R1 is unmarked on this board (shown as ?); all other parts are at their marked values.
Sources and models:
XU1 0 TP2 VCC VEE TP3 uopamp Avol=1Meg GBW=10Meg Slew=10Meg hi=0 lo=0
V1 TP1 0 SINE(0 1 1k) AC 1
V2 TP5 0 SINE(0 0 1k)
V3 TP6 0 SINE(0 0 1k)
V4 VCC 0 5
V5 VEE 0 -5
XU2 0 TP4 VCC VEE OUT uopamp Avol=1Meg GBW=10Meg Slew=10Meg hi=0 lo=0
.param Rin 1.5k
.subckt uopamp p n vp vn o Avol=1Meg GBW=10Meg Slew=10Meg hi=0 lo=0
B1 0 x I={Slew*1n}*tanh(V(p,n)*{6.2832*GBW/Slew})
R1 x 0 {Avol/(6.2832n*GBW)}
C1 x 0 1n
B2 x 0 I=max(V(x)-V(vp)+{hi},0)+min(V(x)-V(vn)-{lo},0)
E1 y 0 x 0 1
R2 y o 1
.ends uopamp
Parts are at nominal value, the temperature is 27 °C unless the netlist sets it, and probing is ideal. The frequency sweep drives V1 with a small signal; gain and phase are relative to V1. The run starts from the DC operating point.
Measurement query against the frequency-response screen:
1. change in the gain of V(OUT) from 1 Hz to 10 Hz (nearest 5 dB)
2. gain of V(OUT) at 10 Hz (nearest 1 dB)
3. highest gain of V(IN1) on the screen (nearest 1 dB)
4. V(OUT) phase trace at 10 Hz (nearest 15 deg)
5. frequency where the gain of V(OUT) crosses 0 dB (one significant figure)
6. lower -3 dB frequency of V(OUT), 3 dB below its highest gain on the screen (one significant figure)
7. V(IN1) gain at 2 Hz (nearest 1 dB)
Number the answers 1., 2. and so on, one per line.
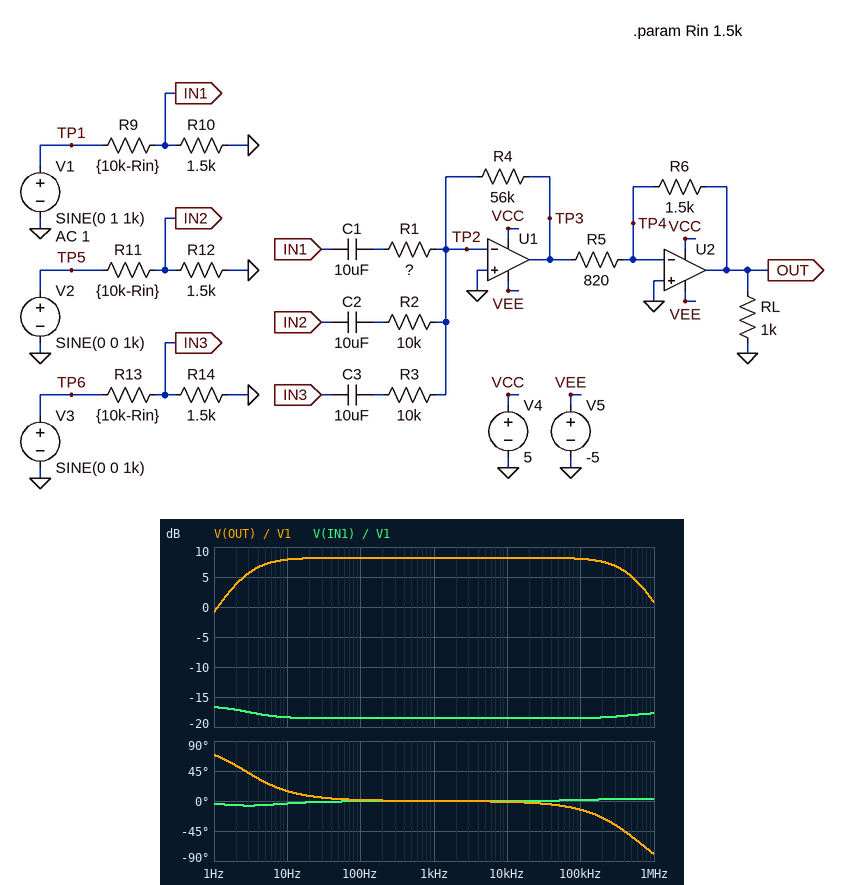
1. 10 dB
2. 8 dB
3. -17 dB
4. 15 deg
5. 1 Hz
6. 3 Hz
7. -17 dB
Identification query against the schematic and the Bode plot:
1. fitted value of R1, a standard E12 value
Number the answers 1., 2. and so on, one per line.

1. 4.7 kΩ
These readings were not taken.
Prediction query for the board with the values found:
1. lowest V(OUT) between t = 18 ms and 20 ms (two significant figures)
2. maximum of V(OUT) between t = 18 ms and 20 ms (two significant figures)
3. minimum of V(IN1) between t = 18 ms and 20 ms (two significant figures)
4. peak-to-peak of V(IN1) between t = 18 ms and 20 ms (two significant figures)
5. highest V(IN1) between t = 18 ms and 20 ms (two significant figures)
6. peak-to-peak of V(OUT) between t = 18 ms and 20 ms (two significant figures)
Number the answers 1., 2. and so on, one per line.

1. -2.6 V
2. 2.6 V
3. -120 mV
4. 240 mV
5. 120 mV
6. 5.1 V
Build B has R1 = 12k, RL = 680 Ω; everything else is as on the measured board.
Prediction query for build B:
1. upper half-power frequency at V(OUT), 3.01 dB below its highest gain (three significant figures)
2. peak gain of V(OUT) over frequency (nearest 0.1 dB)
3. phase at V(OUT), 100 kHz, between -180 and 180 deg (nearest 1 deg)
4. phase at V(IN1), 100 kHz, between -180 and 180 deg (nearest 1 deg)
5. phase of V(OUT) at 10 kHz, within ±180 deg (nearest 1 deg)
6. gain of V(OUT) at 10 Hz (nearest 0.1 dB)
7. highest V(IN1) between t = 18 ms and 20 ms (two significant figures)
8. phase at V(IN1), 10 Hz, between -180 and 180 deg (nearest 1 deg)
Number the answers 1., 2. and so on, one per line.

1. 638 kHz
2. 1.3 dB
3. -10 deg
4. 0 deg
5. -1 deg
6. 1.2 dB
7. 140 mV
8. -1 deg
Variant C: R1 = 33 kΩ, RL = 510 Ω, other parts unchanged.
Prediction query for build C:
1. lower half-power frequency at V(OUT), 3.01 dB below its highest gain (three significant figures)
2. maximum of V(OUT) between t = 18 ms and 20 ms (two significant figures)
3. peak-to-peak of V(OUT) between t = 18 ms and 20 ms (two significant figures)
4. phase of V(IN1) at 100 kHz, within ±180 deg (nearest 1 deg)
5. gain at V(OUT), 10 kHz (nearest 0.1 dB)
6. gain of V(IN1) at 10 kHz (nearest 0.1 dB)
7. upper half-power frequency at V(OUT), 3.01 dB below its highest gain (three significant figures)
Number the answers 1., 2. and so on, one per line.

1. 464 mHz
2. 450 mV
3. 900 mV
4. 0 deg
5. -7.0 dB
6. -16.8 dB
7. 759 kHz
